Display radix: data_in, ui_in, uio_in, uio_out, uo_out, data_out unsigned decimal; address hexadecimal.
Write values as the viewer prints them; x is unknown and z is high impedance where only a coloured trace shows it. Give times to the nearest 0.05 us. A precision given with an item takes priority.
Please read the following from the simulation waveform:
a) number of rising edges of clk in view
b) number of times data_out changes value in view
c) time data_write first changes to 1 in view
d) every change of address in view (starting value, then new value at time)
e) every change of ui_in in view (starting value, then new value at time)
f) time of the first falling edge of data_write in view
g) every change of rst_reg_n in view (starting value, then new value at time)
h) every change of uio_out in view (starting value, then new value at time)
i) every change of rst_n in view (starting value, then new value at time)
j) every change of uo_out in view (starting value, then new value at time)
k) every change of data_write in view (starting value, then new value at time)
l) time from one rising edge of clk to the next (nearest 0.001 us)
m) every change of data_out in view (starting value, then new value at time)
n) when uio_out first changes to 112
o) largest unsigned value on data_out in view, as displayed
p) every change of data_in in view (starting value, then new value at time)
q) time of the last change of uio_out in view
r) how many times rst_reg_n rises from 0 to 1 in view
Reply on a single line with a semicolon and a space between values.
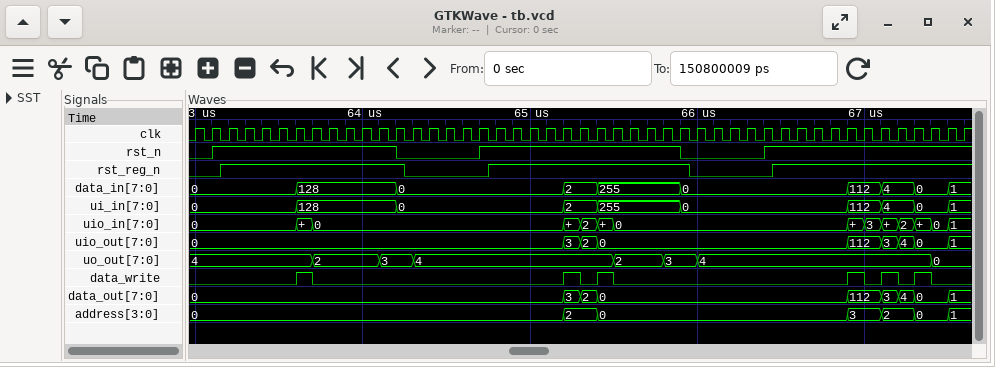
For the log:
47; 8; 63.6 us; 0, 2 at 65.2 us, 0 at 65.4 us, 3 at 66.9 us, 2 at 67.1 us, 0 at 67.3 us, 1 at 67.5 us; 0, 128 at 63.6 us, 0 at 64.2 us, 2 at 65.2 us, 255 at 65.4 us, 0 at 65.9 us, 112 at 66.9 us, 4 at 67.1 us, 0 at 67.3 us, 1 at 67.5 us; 63.7 us; 0, 1 at 63.15 us, 0 at 64.25 us, 1 at 64.75 us, 0 at 65.95 us, 1 at 66.45 us; 0, 3 at 65.2 us, 2 at 65.3 us, 0 at 65.4 us, 112 at 66.9 us, 3 at 67.1 us, 4 at 67.2 us, 0 at 67.3 us, 1 at 67.5 us; 0, 1 at 63.1 us, 0 at 64.2 us, 1 at 64.7 us, 0 at 65.9 us, 1 at 66.4 us; 4, 2 at 63.7 us, 3 at 64.1 us, 4 at 64.3 us, 2 at 65.5 us, 3 at 65.8 us, 4 at 66 us, 0 at 67.4 us; 0, 1 at 63.6 us, 0 at 63.7 us, 1 at 65.2 us, 0 at 65.3 us, 1 at 65.4 us, 0 at 65.5 us, 1 at 66.9 us, 0 at 67 us, 1 at 67.1 us, 0 at 67.2 us, 1 at 67.3 us, 0 at 67.4 us; 0.1 us; 0, 3 at 65.2 us, 2 at 65.3 us, 0 at 65.4 us, 112 at 66.9 us, 3 at 67.1 us, 4 at 67.2 us, 0 at 67.3 us, 1 at 67.5 us; 66.9 us; 112; 0, 128 at 63.6 us, 0 at 64.2 us, 2 at 65.2 us, 255 at 65.4 us, 0 at 65.9 us, 112 at 66.9 us, 4 at 67.1 us, 0 at 67.3 us, 1 at 67.5 us; 67.5 us; 3
